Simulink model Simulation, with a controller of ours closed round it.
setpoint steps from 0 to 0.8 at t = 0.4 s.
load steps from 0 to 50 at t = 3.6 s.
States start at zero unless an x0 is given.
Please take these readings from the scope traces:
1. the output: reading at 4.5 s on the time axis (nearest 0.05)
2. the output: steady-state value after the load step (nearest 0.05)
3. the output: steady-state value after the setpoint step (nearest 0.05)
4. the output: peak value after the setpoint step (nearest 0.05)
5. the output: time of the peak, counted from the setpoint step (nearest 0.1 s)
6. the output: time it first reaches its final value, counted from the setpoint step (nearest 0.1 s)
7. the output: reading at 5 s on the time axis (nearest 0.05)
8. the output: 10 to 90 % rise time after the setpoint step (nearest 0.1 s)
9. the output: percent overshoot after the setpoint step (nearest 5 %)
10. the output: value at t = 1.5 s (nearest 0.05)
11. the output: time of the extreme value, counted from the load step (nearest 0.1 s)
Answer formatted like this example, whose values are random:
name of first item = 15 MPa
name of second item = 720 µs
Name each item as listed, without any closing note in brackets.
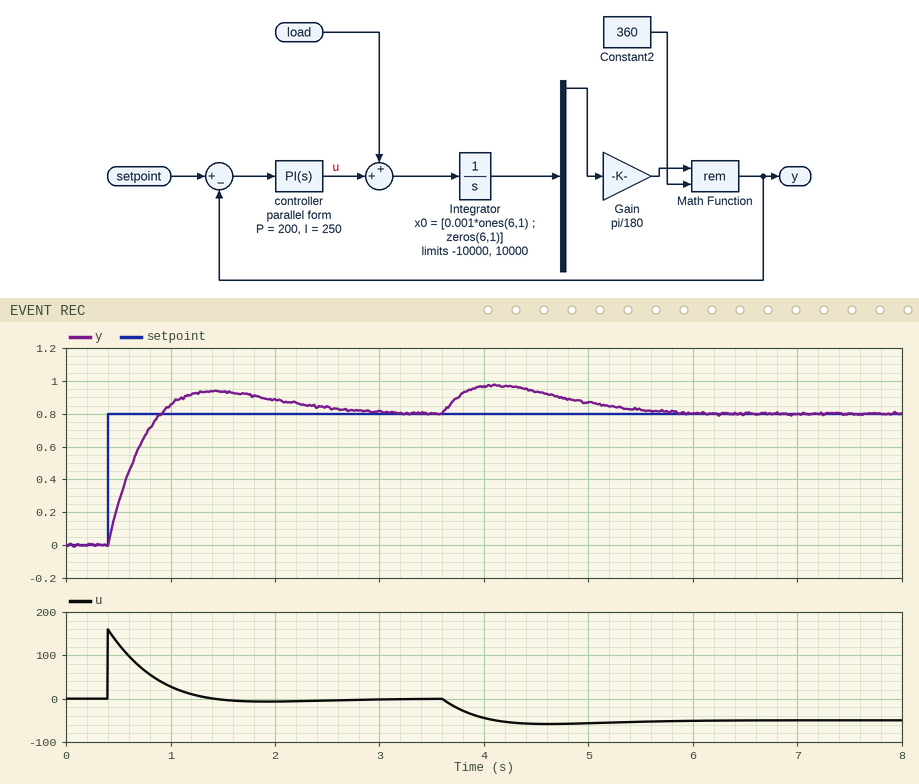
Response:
the output: reading at 4.5 s on the time axis = 0.95
the output: steady-state value after the load step = 0.80
the output: steady-state value after the setpoint step = 0.80
the output: peak value after the setpoint step = 0.95
the output: time of the peak, counted from the setpoint step = 1.0 s
the output: time it first reaches its final value, counted from the setpoint step = 0.5 s
the output: reading at 5 s on the time axis = 0.85
the output: 10 to 90 % rise time after the setpoint step = 0.4 s
the output: percent overshoot after the setpoint step = 15 %
the output: value at t = 1.5 s = 0.95
the output: time of the extreme value, counted from the load step = 0.5 s
